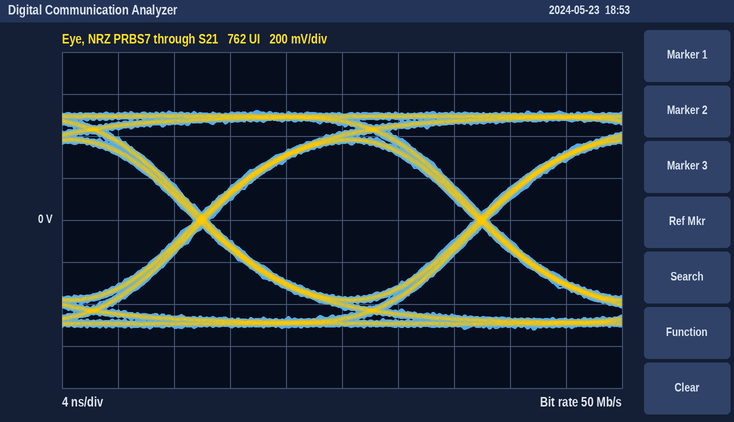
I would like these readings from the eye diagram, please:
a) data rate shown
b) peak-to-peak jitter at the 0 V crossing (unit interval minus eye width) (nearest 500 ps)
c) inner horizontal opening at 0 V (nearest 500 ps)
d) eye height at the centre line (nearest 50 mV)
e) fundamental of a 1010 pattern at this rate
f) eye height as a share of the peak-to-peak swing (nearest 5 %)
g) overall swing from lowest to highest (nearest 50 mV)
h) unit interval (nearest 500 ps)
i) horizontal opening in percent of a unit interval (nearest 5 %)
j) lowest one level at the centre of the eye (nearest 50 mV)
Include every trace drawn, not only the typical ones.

50 Mb/s
1.0 ns
19.0 ns
750 mV
25 MHz
70 %
1.05 V
20.0 ns
95 %
350 mV
